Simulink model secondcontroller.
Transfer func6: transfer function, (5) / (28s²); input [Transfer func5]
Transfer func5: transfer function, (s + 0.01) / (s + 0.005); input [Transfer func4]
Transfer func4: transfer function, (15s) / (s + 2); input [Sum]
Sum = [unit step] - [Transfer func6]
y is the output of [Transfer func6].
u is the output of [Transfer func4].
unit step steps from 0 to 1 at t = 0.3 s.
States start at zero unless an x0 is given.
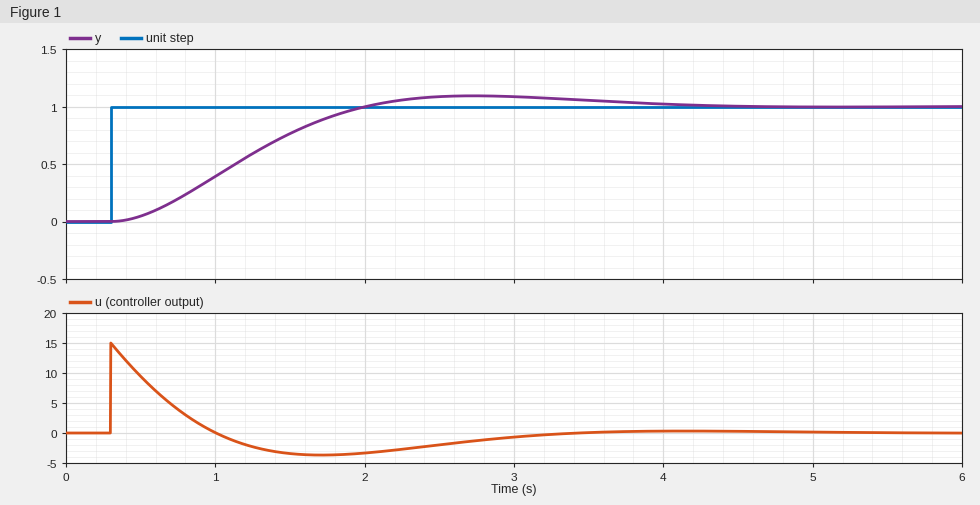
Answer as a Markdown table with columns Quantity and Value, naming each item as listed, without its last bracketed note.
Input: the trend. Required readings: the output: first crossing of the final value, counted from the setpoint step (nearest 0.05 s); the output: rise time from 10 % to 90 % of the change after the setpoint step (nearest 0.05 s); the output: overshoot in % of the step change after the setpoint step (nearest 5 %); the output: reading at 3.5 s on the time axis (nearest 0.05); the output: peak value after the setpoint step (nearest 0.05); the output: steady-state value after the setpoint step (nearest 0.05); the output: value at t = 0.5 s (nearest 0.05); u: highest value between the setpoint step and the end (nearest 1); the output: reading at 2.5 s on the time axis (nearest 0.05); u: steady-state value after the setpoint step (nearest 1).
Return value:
| Quantity | Value |
|---|---|
| the output: first crossing of the final value, counted from the setpoint step | 1.70 s |
| the output: rise time from 10 % to 90 % of the change after the setpoint step | 1.15 s |
| the output: overshoot in % of the step change after the setpoint step | 10 % |
| the output: reading at 3.5 s on the time axis | 1.05 |
| the output: peak value after the setpoint step | 1.10 |
| the output: steady-state value after the setpoint step | 1.00 |
| the output: value at t = 0.5 s | 0.05 |
| u: highest value between the setpoint step and the end | 15 |
| the output: reading at 2.5 s on the time axis | 1.10 |
| u: steady-state value after the setpoint step | 0 |
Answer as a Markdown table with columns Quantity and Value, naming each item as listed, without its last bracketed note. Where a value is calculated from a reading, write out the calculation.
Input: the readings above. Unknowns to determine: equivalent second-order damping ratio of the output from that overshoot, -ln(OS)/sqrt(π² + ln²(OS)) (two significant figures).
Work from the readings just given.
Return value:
| Quantity | Value |
|---|---|
| equivalent second-order damping ratio of the output from that overshoot, -ln(OS)/sqrt(π² + ln²(OS)) | ln(0.1) = -2.303; 2.303 / sqrt(9.870 + 5.302) = 0.59 |
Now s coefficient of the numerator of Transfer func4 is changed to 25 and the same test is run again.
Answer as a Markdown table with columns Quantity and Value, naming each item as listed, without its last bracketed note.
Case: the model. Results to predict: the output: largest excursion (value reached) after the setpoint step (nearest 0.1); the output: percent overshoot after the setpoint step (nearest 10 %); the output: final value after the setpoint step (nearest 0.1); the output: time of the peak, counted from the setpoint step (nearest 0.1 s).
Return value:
| Quantity | Value |
|---|---|
| the output: largest excursion (value reached) after the setpoint step | 1.2 |
| the output: percent overshoot after the setpoint step | 20 % |
| the output: final value after the setpoint step | 1.0 |
| the output: time of the peak, counted from the setpoint step | 1.7 s |
